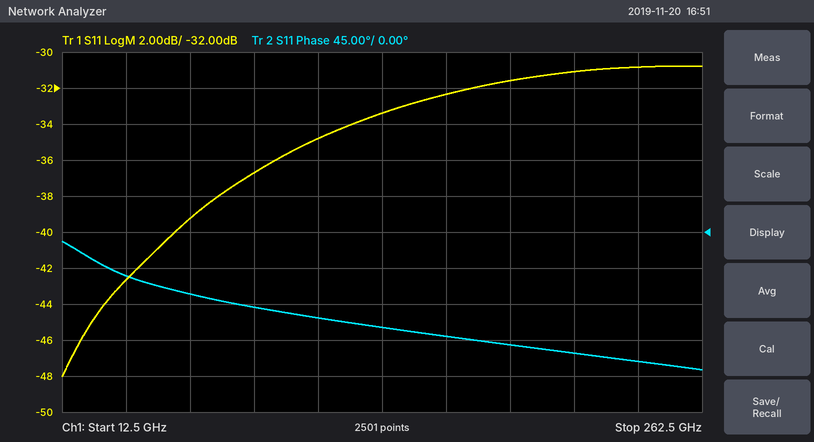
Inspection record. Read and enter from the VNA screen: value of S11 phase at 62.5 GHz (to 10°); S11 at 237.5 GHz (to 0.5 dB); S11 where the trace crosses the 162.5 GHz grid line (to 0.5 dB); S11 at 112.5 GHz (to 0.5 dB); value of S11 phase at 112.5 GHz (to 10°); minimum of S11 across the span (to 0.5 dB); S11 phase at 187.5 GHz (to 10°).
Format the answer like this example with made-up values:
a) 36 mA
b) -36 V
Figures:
a) -80°
b) -31.0 dB
c) -32.5 dB
d) -35.0 dB
e) -110°
f) -48.0 dB
g) -140°
